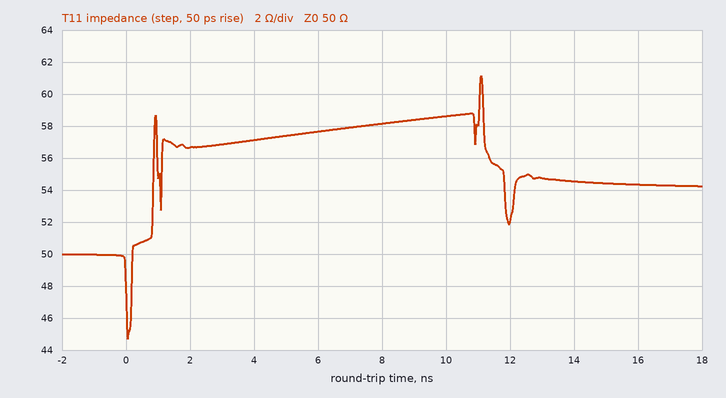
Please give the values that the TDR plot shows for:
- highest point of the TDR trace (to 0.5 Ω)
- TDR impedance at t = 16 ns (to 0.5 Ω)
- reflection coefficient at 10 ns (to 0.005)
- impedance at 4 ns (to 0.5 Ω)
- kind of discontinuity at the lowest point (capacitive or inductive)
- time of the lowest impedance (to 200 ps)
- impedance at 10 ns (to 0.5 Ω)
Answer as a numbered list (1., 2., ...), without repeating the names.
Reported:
1. 61.0 Ω
2. 54.5 Ω
3. +0.080
4. 57.0 Ω
5. capacitive
6. 0.0 ns
7. 58.5 Ω
